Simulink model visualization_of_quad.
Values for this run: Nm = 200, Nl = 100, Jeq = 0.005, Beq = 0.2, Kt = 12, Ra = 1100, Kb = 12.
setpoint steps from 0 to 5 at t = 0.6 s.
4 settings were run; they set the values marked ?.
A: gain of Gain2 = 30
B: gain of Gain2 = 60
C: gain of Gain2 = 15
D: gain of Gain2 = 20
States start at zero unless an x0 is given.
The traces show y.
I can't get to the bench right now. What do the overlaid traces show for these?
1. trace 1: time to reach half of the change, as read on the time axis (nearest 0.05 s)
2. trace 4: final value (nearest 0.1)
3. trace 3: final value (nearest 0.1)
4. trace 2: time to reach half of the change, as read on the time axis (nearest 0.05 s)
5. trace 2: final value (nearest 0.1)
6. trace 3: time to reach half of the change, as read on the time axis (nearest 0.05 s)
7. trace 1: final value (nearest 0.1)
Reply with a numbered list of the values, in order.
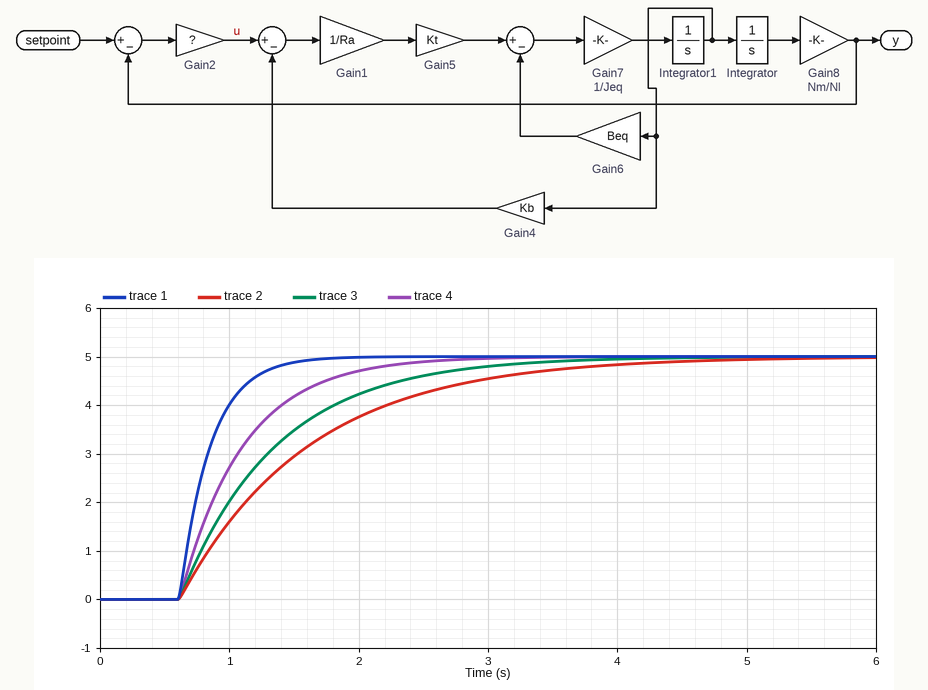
1. 0.80 s
2. 5.0
3. 5.0
4. 1.30 s
5. 5.0
6. 1.15 s
7. 5.0
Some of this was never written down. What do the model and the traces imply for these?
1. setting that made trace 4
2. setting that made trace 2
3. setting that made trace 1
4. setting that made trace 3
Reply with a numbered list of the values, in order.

1. A
2. C
3. B
4. D
